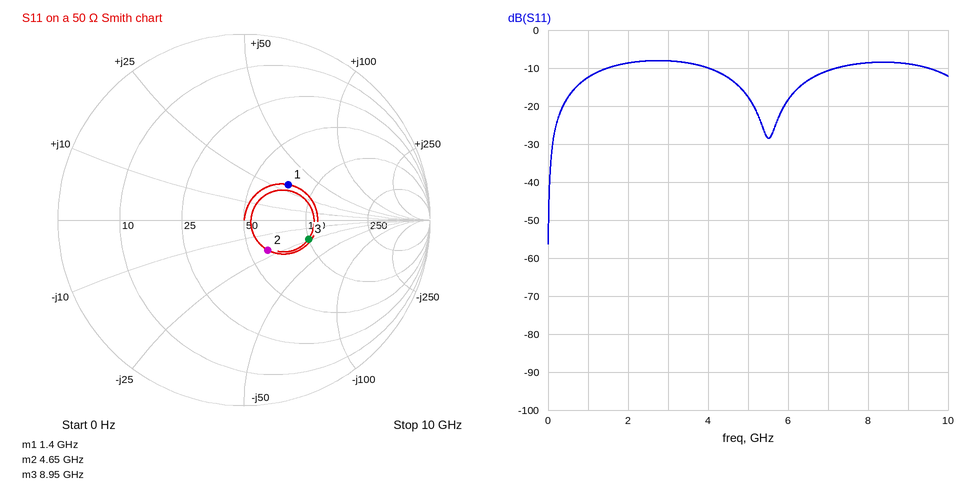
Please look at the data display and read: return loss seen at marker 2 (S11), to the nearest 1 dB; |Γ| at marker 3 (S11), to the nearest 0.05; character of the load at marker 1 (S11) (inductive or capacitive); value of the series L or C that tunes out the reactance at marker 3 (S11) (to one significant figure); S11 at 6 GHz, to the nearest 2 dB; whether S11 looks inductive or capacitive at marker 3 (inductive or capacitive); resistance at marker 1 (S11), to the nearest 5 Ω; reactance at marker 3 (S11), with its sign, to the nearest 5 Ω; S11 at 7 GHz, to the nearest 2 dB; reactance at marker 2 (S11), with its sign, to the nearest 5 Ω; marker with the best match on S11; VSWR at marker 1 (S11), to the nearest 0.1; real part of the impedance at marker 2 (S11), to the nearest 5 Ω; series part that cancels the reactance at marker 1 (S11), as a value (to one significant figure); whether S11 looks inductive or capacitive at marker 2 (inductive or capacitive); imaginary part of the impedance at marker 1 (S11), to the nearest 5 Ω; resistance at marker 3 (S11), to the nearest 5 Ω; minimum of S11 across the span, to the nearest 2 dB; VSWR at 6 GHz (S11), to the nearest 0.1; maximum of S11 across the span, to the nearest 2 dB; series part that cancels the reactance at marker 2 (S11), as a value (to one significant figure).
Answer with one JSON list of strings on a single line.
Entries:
["14 dB", "0.35", "inductive", "400 pH", "-18 dB", "capacitive", "75 Ω", "-25 Ω", "-10 dB", "-20 Ω", "marker 2", "1.9", "60 Ω", "4 pF", "capacitive", "+30 Ω", "100 Ω", "-56 dB", "1.3", "-8 dB", "700 pH"]
